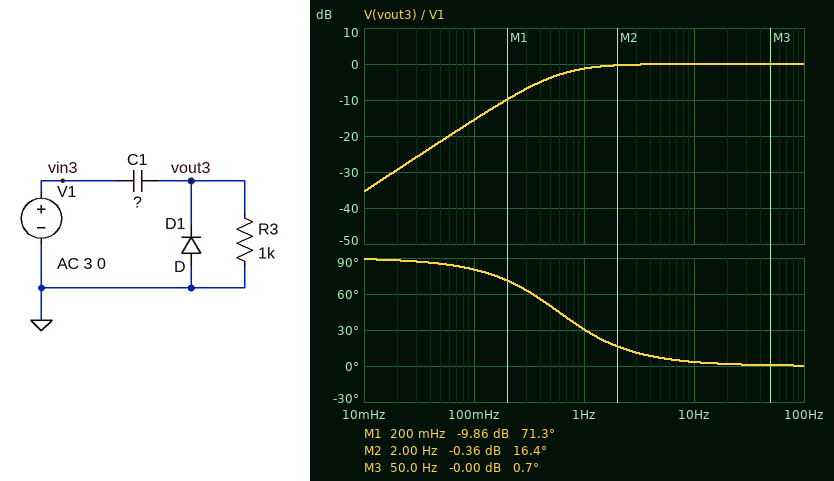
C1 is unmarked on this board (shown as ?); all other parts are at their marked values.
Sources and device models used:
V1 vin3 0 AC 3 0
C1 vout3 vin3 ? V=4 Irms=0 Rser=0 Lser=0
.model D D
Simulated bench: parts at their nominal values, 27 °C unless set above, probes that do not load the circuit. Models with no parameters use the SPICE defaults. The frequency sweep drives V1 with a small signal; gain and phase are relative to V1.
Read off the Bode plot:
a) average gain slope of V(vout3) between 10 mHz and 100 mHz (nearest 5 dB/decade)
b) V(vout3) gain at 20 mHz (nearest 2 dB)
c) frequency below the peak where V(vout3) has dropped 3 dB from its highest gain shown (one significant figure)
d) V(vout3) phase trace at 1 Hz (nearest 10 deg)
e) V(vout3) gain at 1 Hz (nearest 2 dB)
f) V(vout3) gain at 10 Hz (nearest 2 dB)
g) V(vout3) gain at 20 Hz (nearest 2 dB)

20 dB/decade
-30 dB
600 mHz
30 deg
-2 dB
0 dB
0 dB
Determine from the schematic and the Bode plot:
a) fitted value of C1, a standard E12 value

270 µF
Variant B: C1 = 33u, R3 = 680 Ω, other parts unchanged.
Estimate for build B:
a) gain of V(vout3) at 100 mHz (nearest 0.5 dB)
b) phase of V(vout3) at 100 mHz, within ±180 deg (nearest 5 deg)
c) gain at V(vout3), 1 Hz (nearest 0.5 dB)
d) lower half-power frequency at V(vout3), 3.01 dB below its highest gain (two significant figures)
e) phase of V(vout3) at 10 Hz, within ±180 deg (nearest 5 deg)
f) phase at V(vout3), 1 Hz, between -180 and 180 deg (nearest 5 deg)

-37.0 dB
90 deg
-17.0 dB
7.1 Hz
35 deg
80 deg
